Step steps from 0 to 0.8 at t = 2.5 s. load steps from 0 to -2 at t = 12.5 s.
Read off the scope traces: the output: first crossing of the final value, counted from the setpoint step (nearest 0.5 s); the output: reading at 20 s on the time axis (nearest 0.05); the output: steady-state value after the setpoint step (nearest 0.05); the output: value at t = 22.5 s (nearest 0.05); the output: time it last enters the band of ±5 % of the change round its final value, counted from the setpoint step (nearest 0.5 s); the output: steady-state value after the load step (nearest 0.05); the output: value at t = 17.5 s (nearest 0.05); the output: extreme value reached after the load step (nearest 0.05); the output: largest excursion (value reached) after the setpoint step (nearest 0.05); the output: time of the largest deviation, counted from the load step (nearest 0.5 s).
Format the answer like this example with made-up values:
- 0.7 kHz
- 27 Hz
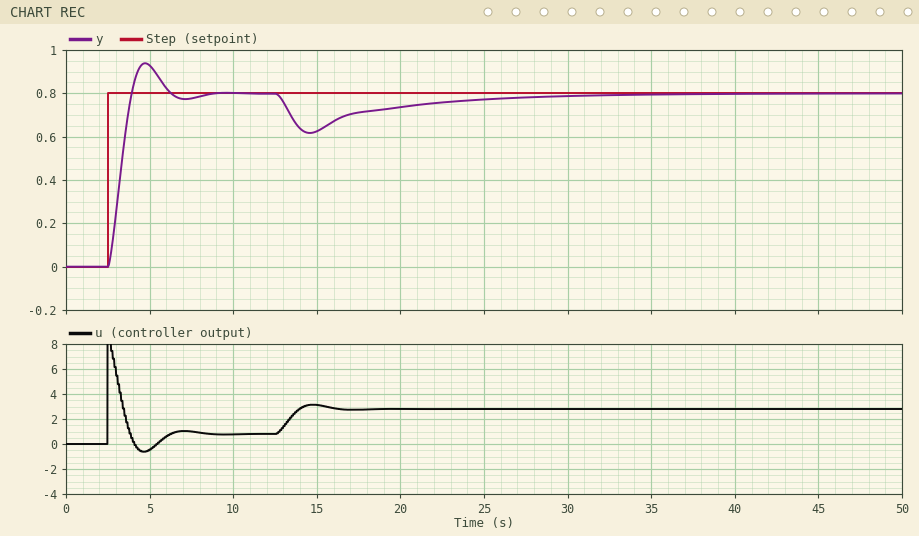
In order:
- 1.5 s
- 0.75
- 0.80
- 0.75
- 3.5 s
- 0.80
- 0.70
- 0.60
- 0.95
- 2.0 s
